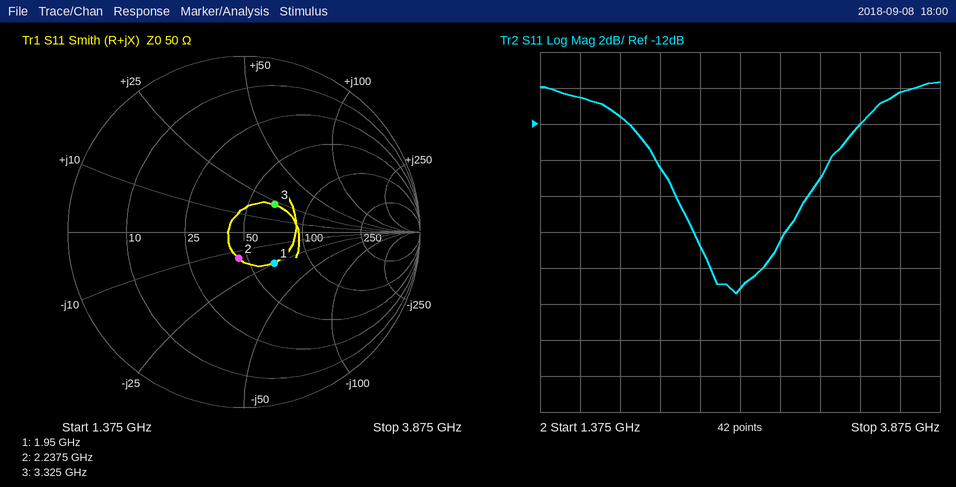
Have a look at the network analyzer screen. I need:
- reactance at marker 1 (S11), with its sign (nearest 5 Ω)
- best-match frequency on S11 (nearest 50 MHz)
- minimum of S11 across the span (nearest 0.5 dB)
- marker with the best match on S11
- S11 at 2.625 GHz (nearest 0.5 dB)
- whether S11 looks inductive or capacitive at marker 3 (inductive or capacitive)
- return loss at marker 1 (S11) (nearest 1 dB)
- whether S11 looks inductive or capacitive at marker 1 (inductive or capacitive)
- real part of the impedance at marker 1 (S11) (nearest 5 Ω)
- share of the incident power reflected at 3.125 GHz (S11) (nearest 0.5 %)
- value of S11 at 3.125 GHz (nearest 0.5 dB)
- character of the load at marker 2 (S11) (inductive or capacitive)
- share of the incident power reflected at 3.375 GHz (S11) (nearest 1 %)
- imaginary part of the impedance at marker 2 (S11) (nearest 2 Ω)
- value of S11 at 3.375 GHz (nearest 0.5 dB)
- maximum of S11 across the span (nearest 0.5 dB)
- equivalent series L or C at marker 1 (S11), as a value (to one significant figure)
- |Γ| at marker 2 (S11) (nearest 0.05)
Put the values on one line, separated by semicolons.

-25 Ω; 2.60 GHz; -21.5 dB; marker 2; -21.0 dB; inductive; 12 dB; capacitive; 65 Ω; 3.0 %; -15.0 dB; capacitive; 6 %; -14 Ω; -12.0 dB; -9.5 dB; 3 pF; 0.15
